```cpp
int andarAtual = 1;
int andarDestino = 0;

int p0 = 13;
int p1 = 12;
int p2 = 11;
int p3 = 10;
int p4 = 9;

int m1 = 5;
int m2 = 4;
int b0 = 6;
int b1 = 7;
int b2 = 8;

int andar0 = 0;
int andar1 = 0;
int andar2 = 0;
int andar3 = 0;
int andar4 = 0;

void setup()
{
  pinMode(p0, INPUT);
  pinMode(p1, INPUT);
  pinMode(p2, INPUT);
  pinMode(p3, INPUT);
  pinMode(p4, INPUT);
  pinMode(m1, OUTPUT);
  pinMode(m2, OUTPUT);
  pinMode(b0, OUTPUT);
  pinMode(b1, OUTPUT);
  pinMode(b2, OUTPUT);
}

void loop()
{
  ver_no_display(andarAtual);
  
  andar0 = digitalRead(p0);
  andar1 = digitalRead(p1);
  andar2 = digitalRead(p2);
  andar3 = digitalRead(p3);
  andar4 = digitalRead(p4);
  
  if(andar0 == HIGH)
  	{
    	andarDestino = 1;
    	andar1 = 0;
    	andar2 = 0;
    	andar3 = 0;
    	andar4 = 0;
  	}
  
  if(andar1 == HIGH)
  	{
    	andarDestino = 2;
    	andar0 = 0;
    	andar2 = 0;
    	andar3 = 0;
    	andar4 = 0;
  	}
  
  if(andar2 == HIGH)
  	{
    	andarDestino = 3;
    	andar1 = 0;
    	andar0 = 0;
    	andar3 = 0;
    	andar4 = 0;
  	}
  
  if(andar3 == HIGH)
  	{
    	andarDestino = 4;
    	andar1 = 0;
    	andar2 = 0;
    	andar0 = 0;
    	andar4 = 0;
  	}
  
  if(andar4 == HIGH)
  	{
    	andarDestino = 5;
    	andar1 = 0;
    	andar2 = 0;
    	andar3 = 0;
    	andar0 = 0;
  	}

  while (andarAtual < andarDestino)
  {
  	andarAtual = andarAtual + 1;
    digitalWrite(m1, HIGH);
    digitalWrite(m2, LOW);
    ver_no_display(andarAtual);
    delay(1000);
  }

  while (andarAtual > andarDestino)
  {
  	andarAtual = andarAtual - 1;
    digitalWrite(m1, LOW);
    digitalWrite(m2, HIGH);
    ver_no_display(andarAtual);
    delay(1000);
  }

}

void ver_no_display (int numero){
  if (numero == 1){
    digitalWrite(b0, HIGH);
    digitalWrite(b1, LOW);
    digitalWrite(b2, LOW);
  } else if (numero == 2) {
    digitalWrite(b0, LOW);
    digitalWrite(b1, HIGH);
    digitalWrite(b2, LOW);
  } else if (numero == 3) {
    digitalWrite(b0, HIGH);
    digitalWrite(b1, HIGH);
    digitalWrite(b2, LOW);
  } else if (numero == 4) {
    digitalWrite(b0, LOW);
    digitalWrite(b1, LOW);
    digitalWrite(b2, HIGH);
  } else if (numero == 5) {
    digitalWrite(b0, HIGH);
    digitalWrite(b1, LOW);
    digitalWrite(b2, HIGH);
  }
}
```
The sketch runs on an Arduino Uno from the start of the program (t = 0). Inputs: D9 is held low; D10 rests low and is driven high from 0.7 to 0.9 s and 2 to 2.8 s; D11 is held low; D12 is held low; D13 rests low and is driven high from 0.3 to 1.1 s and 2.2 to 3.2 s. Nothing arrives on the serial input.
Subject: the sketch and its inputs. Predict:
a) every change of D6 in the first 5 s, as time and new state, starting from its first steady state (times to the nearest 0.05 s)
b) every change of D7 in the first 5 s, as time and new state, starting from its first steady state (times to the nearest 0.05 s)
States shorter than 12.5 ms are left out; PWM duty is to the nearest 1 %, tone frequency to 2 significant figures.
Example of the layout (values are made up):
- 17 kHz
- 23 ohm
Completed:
- 0 s high; 2 s low; 3 s high; 4 s low
- 0 s low; 2 s high; 4 s low
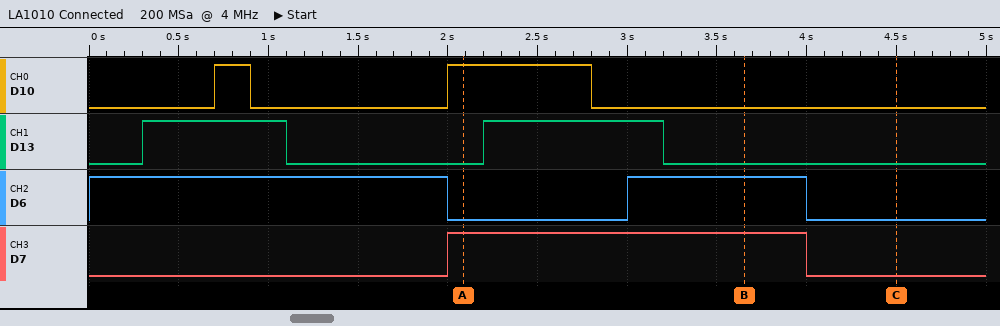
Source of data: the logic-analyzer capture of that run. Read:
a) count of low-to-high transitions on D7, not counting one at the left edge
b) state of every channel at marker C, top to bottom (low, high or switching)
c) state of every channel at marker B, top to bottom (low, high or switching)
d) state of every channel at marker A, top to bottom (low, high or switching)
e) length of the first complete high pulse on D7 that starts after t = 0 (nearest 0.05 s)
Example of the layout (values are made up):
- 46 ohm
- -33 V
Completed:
- 1
- D10 low, D13 low, D6 low, D7 low
- D10 low, D13 low, D6 high, D7 high
- D10 high, D13 low, D6 low, D7 high
- 2.00 s
